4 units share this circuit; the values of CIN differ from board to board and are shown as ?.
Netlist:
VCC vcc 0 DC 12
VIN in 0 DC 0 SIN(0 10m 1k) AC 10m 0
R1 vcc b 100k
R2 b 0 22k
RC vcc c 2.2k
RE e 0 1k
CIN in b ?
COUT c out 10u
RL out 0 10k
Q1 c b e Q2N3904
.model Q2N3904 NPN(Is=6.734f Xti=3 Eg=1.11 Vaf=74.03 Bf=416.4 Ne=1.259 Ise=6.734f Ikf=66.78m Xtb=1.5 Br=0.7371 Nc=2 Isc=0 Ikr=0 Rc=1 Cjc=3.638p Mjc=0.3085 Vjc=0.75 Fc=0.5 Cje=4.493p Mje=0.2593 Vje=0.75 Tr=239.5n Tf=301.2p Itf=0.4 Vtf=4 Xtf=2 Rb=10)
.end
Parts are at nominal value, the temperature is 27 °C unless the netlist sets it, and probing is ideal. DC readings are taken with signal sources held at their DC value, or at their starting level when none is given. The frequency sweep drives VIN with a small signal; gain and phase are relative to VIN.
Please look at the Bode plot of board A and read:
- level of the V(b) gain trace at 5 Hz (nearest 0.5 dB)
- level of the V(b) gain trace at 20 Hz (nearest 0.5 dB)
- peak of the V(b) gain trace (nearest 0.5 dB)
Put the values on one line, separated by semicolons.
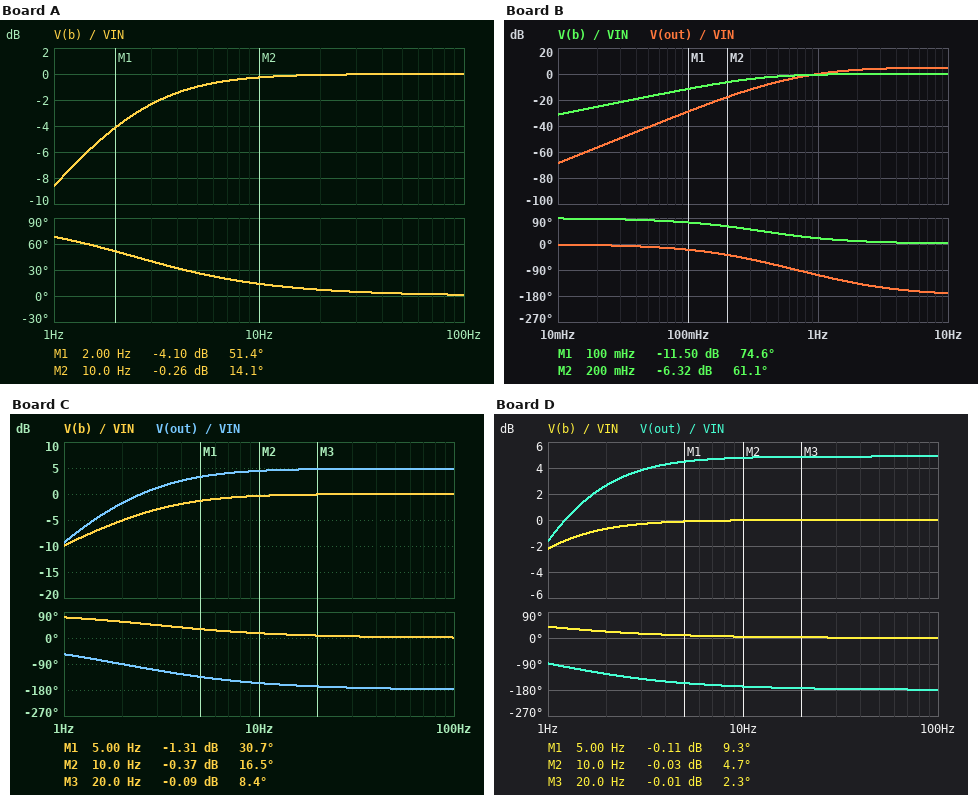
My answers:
-1.0 dB; 0 dB; 0 dB
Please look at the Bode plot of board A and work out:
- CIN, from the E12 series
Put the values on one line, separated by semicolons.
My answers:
3.9 µF
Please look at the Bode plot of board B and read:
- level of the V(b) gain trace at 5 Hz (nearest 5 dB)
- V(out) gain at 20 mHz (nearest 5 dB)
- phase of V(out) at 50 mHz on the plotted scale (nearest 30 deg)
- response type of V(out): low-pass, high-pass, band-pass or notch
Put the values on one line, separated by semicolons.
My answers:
0 dB; -55 dB; 0 deg; high-pass
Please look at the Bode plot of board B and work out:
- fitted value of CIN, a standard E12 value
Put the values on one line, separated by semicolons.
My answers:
27 µF
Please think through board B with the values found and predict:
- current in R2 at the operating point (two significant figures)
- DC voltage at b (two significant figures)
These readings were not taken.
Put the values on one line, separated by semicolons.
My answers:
91 µA; 2.0 V
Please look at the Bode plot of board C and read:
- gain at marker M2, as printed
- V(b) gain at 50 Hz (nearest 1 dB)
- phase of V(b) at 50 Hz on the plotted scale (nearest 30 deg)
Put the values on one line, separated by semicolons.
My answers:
-0.37 dB; 0 dB; 0 deg
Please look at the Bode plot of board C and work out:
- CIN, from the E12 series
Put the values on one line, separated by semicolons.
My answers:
3.3 µF
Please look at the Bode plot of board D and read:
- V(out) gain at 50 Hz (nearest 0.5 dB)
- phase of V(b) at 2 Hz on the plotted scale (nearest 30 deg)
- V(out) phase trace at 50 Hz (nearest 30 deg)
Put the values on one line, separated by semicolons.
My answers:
5.0 dB; 30 deg; -180 deg
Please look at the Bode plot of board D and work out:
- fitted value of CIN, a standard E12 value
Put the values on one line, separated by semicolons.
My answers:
12 µF
